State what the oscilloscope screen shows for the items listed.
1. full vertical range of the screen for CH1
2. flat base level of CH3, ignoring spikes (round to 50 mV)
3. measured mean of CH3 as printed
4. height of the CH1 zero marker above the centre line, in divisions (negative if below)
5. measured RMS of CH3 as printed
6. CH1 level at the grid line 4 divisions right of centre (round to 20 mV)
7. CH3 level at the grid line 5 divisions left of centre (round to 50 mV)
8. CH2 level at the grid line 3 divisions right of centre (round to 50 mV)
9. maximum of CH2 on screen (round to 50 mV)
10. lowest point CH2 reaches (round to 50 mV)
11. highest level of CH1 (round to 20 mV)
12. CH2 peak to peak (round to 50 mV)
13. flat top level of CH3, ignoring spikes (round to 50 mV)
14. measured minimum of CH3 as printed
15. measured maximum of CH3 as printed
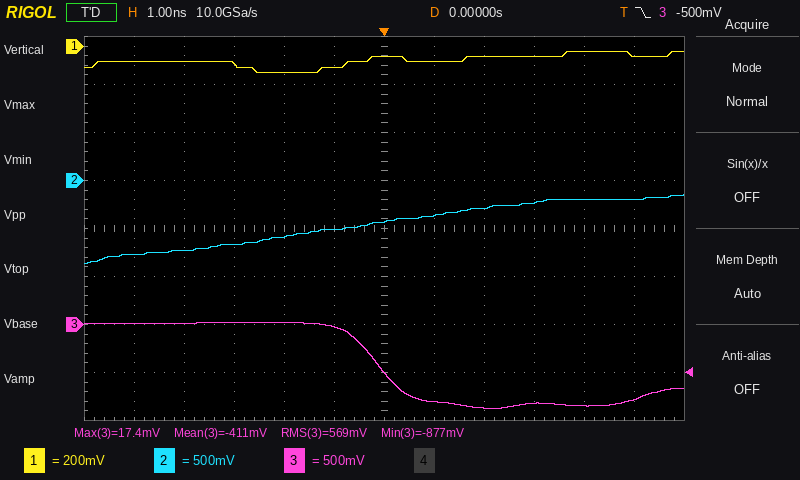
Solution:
1.6 V
-850 mV
-411 mV
+3.8 div
569 mV
-20 mV
0 mV
-250 mV
-150 mV
-850 mV
-20 mV
700 mV
0 mV
-877 mV
17.4 mV
